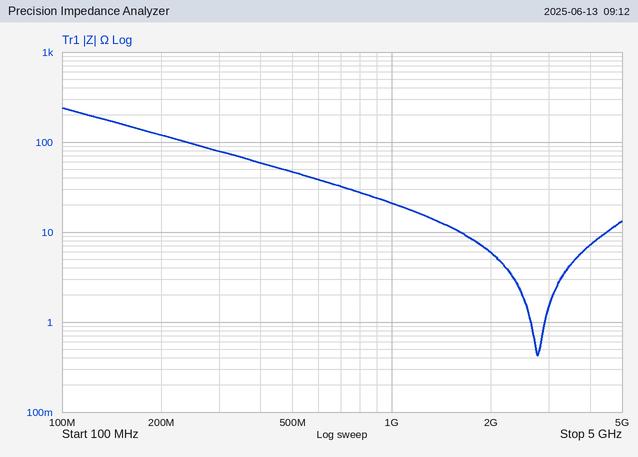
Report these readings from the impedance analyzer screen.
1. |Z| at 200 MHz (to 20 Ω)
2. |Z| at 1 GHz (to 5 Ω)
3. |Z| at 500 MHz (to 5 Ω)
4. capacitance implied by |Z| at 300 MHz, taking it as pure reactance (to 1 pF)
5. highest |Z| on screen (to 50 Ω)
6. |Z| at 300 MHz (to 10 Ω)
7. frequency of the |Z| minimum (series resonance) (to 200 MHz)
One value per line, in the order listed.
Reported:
120 Ω
20 Ω
45 Ω
7 pF
250 Ω
80 Ω
2.8 GHz
